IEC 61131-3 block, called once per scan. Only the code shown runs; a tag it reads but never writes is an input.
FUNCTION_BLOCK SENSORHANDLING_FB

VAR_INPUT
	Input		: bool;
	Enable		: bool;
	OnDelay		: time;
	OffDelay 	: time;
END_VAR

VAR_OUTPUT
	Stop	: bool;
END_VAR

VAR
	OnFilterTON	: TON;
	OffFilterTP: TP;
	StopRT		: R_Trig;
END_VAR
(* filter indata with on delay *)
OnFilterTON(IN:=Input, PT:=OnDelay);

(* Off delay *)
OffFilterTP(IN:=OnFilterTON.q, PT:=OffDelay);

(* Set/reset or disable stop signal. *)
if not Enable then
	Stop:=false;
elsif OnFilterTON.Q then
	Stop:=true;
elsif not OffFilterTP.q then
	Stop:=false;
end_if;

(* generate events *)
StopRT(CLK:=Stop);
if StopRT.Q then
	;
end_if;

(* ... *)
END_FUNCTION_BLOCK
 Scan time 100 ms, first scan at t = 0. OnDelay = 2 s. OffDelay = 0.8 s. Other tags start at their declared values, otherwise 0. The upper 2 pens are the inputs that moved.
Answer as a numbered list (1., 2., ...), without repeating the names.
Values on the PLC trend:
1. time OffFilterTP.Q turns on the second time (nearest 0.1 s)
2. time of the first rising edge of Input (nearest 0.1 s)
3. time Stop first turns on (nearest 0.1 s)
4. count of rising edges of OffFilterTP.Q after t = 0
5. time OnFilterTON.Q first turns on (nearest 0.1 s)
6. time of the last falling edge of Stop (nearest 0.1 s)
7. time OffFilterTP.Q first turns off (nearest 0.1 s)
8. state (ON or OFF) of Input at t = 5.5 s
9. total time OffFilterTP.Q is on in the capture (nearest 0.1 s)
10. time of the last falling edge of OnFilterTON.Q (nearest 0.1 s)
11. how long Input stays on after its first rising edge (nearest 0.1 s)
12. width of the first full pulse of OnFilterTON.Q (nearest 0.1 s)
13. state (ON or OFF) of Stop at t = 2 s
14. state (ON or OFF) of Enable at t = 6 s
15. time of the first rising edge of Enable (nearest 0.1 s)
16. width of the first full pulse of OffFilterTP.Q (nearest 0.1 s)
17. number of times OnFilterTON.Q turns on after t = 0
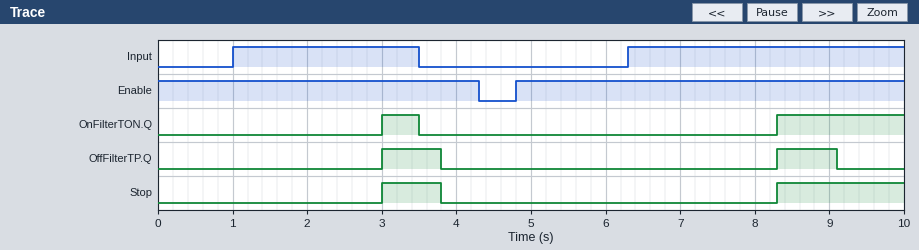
1. 8.3 s
2. 1.0 s
3. 3.0 s
4. 2
5. 3.0 s
6. 3.8 s
7. 3.8 s
8. OFF
9. 1.6 s
10. 3.5 s
11. 2.5 s
12. 0.5 s
13. OFF
14. ON
15. 4.8 s
16. 0.8 s
17. 2
